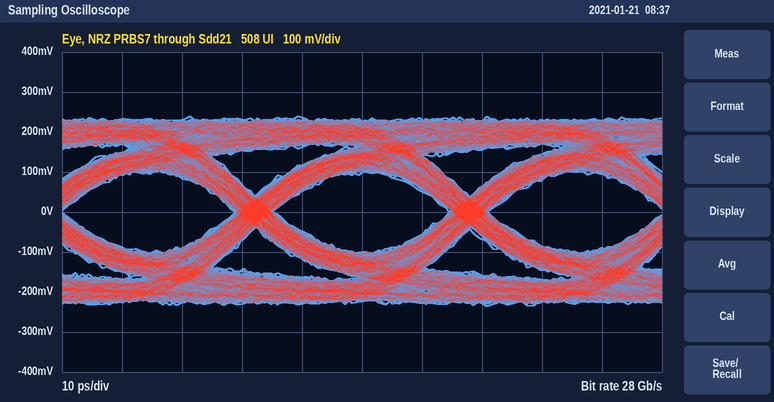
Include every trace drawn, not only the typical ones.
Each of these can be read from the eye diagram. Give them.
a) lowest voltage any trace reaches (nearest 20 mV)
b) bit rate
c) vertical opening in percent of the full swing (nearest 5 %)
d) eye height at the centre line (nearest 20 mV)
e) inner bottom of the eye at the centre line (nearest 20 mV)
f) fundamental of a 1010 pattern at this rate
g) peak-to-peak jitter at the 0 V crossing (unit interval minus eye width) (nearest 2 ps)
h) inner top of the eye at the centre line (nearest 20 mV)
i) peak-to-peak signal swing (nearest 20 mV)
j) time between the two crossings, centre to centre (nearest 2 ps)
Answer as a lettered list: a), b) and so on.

a) -240 mV
b) 28 Gb/s
c) 40 %
d) 200 mV
e) -100 mV
f) 14 GHz
g) 6 ps
h) 100 mV
i) 480 mV
j) 36 ps
